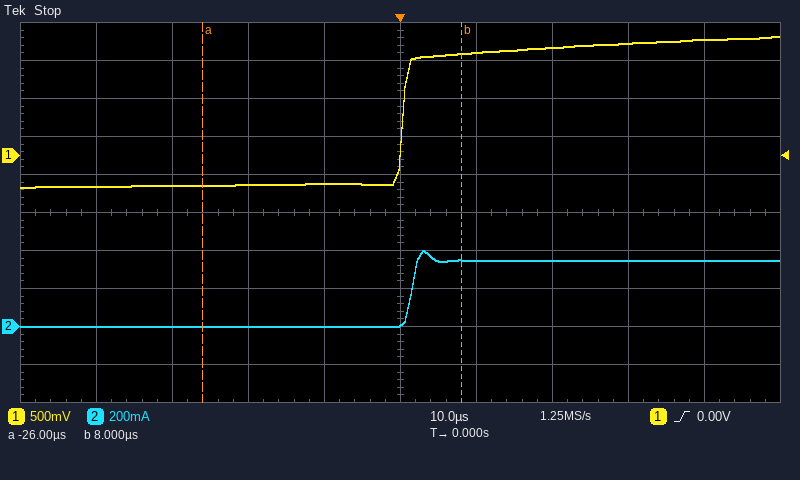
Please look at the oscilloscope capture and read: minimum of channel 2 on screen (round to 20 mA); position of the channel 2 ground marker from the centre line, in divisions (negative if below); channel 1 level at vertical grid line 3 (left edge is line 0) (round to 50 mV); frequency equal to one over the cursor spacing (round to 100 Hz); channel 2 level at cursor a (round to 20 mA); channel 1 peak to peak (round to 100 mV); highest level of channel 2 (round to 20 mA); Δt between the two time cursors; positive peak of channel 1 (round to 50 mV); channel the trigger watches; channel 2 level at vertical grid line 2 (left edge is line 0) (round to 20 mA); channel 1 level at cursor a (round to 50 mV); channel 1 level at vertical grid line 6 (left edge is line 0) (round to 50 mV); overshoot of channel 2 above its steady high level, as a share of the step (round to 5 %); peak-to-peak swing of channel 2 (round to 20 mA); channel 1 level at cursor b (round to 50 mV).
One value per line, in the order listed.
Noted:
0 mA
-3.0 div
-400 mV
29.4 kHz
0 mA
2.00 V
400 mA
34 µs
1.55 V
channel 1
0 mA
-400 mV
1.35 V
15 %
400 mA
1.35 V
